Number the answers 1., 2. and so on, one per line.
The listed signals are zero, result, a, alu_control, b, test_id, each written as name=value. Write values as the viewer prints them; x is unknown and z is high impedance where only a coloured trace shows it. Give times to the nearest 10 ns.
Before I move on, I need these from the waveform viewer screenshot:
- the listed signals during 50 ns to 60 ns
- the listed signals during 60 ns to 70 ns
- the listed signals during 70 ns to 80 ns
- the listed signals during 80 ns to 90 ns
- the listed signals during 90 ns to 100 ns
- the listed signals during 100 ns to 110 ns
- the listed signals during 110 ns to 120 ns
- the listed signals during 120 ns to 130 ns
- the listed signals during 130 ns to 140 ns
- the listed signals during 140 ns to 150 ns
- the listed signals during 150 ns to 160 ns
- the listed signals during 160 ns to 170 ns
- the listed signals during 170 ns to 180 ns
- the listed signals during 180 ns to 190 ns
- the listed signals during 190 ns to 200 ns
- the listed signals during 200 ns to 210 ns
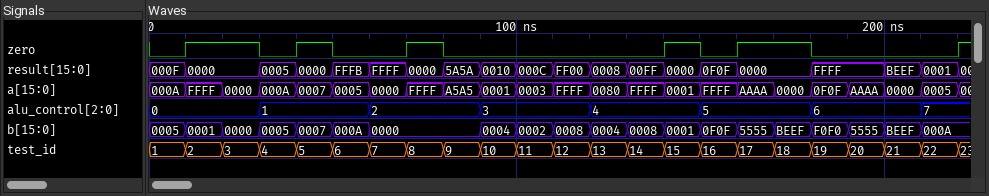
1. zero=0, result=FFFB, a=0005, alu_control=1, b=000A, test_id=6
2. zero=0, result=FFFF, a=0000, alu_control=2, b=0000, test_id=7
3. zero=1, result=0000, a=FFFF, alu_control=2, b=0000, test_id=8
4. zero=0, result=5A5A, a=A5A5, alu_control=2, b=0000, test_id=9
5. zero=0, result=0010, a=0001, alu_control=3, b=0004, test_id=10
6. zero=0, result=000C, a=0003, alu_control=3, b=0002, test_id=11
7. zero=0, result=FF00, a=FFFF, alu_control=3, b=0008, test_id=12
8. zero=0, result=0008, a=0080, alu_control=4, b=0004, test_id=13
9. zero=0, result=00FF, a=FFFF, alu_control=4, b=0008, test_id=14
10. zero=1, result=0000, a=0001, alu_control=4, b=0001, test_id=15
11. zero=0, result=0F0F, a=FFFF, alu_control=5, b=0F0F, test_id=16
12. zero=1, result=0000, a=AAAA, alu_control=5, b=5555, test_id=17
13. zero=1, result=0000, a=0000, alu_control=5, b=BEEF, test_id=18
14. zero=0, result=FFFF, a=0F0F, alu_control=6, b=F0F0, test_id=19
15. zero=0, result=FFFF, a=AAAA, alu_control=6, b=5555, test_id=20
16. zero=0, result=BEEF, a=0000, alu_control=6, b=BEEF, test_id=21
